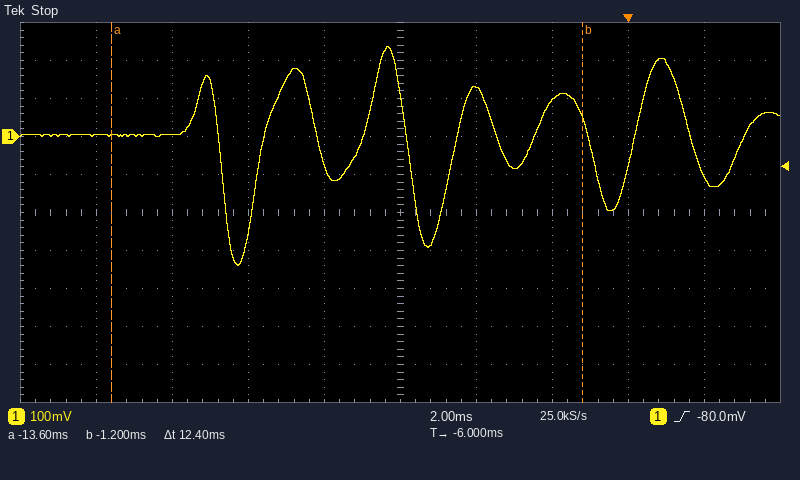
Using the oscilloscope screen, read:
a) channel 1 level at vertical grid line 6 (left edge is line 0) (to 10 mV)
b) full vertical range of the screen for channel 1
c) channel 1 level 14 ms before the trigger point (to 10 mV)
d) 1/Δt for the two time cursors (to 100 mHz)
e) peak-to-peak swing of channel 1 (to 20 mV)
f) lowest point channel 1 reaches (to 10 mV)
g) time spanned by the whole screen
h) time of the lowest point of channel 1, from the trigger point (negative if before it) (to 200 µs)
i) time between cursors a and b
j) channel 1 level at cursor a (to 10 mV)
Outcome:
130 mV
1 V
0 mV
80.6 Hz
580 mV
-340 mV
20 ms
-10.2 ms
12.4 ms
0 mV
